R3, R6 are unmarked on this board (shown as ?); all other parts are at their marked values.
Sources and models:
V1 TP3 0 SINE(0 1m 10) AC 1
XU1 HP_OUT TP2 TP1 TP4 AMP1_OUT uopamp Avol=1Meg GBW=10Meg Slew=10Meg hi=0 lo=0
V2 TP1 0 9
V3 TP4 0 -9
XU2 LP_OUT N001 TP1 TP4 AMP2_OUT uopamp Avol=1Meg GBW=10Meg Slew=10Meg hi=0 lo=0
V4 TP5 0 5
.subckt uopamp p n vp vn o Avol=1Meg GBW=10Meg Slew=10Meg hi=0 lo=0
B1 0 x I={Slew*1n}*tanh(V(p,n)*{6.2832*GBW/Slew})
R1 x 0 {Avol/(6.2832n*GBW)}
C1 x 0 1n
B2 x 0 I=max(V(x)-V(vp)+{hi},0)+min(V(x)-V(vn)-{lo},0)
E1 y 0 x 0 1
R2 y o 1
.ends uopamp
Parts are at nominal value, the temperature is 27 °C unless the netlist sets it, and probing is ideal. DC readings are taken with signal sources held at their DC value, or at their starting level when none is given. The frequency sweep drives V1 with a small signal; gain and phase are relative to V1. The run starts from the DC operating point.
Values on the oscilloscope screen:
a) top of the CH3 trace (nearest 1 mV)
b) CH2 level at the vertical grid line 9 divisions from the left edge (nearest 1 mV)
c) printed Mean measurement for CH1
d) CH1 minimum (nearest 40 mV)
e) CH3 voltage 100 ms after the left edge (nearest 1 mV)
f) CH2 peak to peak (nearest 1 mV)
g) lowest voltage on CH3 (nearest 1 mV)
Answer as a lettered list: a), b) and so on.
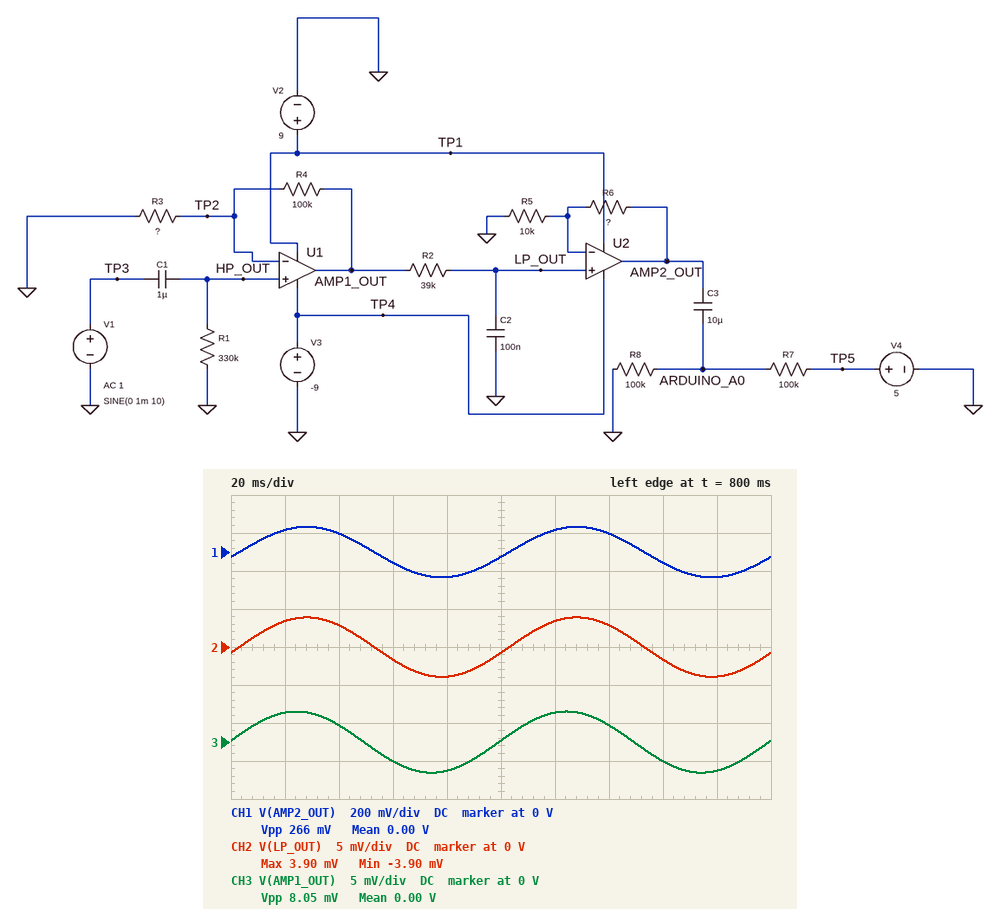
a) 4 mV
b) -4 mV
c) 0.00 V
d) -120 mV
e) 0 V
f) 8 mV
g) -4 mV
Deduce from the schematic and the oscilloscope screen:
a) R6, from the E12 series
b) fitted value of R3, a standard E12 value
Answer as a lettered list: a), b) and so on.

a) 330 kΩ
b) 33 kΩ
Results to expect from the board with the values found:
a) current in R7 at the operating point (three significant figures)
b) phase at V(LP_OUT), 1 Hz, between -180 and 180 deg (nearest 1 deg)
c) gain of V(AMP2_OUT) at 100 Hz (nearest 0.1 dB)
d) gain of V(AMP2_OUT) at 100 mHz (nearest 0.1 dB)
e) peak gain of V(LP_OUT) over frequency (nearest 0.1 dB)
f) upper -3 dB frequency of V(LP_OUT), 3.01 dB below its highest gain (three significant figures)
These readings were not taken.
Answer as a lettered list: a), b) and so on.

a) 25.0 µA
b) 24 deg
c) 34.3 dB
d) 28.9 dB
e) 12.0 dB
f) 41.8 Hz
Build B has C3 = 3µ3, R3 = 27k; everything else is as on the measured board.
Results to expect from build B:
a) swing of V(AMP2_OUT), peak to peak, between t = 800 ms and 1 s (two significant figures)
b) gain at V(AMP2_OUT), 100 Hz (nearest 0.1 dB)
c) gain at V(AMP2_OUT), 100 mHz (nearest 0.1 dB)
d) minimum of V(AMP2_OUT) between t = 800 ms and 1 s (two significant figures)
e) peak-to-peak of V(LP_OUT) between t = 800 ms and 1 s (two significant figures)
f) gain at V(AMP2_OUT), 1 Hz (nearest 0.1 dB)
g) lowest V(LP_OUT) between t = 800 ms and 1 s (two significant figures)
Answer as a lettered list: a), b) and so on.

a) 310 mV
b) 35.6 dB
c) 30.2 dB
d) -160 mV
e) 9.1 mV
f) 43.2 dB
g) -4.6 mV
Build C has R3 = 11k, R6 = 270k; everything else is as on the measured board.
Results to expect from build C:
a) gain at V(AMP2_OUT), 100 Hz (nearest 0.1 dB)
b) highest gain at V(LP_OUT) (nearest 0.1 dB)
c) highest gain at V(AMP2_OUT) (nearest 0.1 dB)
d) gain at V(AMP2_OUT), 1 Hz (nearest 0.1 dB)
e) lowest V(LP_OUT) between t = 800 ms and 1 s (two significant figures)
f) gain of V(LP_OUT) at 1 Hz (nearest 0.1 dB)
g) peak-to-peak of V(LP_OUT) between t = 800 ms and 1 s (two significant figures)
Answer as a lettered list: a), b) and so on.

a) 40.6 dB
b) 20.0 dB
c) 48.9 dB
d) 48.1 dB
e) -9.8 mV
f) 19.2 dB
g) 20 mV
